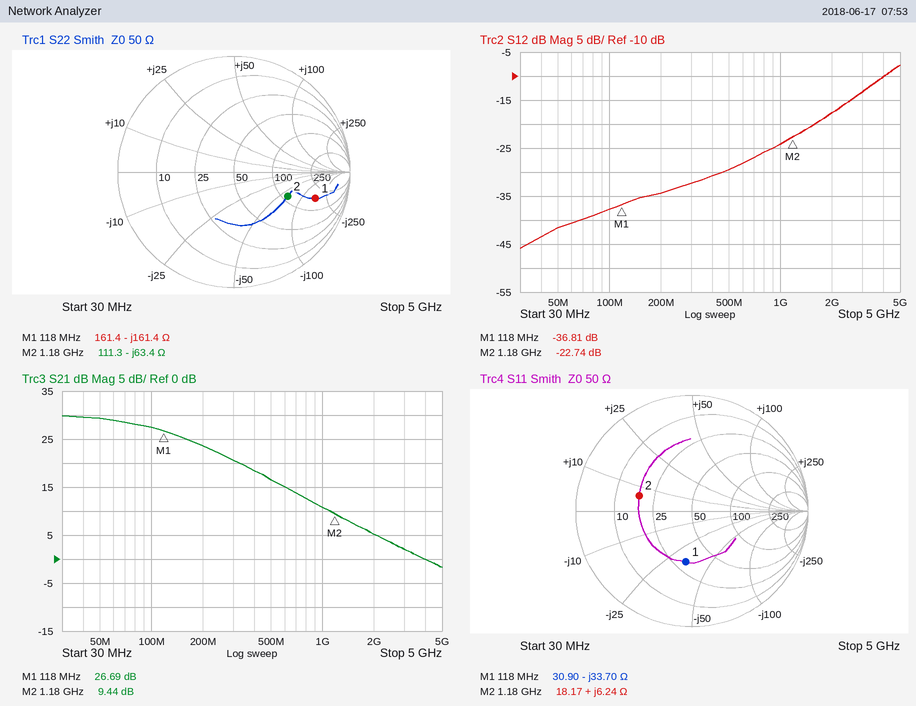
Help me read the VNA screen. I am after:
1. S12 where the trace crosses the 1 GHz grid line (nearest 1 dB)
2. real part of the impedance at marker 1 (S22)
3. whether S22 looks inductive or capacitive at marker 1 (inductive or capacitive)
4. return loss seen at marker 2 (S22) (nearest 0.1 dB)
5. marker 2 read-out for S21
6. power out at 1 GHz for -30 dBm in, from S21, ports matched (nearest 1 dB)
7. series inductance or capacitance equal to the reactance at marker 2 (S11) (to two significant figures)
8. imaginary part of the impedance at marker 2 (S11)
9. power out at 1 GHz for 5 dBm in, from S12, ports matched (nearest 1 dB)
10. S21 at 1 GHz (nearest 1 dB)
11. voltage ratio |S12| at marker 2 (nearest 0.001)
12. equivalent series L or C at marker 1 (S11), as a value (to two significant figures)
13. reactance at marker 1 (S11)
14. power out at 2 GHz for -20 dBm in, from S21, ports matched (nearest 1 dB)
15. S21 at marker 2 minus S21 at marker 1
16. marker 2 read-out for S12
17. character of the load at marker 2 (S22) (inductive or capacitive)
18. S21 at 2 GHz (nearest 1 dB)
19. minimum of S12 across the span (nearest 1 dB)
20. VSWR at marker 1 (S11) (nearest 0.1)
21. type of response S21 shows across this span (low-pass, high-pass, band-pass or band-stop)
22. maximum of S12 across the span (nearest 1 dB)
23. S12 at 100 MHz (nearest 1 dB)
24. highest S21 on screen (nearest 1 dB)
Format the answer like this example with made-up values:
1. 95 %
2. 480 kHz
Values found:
1. -24 dB
2. 161.4 Ω
3. capacitive
4. 5.9 dB
5. 9.44 dB
6. -19 dBm
7. 840 pH
8. +6.24 Ω
9. -19 dBm
10. 11 dB
11. 0.073
12. 40 pF
13. -33.70 Ω
14. -15 dBm
15. -17.25 dB
16. -22.74 dB
17. capacitive
18. 5 dB
19. -46 dB
20. 2.6
21. low-pass
22. -8 dB
23. -38 dB
24. 30 dB
